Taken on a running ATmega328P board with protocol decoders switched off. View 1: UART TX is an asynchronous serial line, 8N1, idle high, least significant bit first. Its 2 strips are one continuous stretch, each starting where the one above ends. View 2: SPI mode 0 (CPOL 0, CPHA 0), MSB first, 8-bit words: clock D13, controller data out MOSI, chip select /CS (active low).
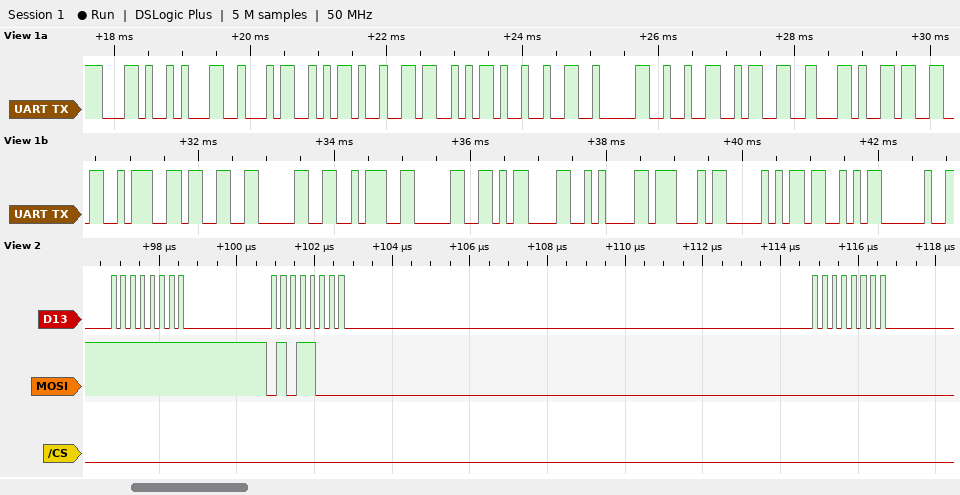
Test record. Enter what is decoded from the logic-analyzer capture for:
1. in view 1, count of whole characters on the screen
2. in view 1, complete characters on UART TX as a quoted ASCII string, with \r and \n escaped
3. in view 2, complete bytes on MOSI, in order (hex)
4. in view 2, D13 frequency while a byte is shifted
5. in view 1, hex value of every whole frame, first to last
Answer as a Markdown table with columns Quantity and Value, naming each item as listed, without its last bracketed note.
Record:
| Quantity | Value |
|---|---|
| in view 1, count of whole characters on the screen | 23 |
| in view 1, complete characters on UART TX as a quoted ASCII string, with \r and \n escaped | ",14-6-2023,3:30:0\r\nGPS " |
| in view 2, complete bytes on MOSI, in order | FF 58 00 |
| in view 2, D13 frequency while a byte is shifted | 4 MHz |
| in view 1, hex value of every whole frame, first to last | 0x2C 0x31 0x34 0x2D 0x36 0x2D 0x32 0x30 0x32 0x33 0x2C 0x33 0x3A 0x33 0x30 0x3A 0x30 0x0D 0x0A 0x47 0x50 0x53 0x20 |
